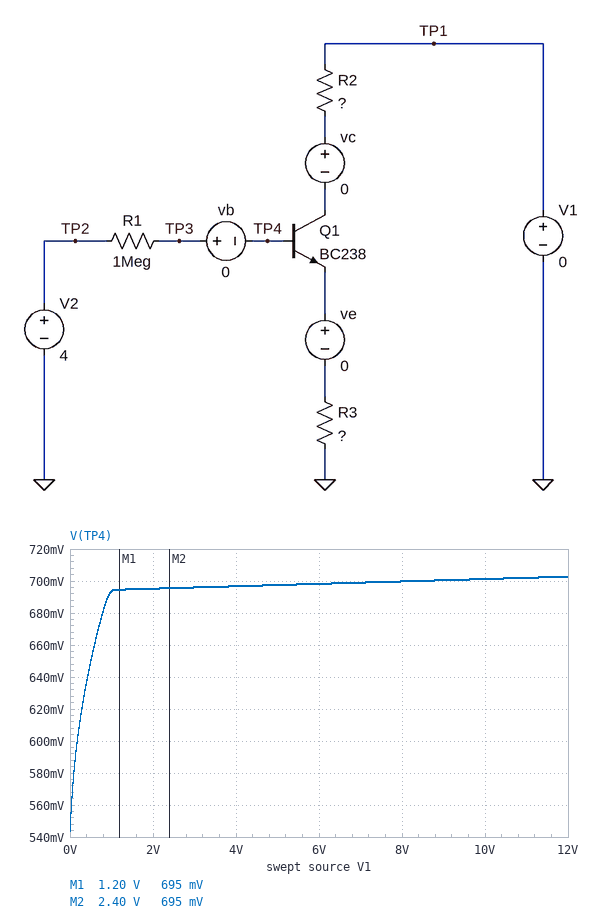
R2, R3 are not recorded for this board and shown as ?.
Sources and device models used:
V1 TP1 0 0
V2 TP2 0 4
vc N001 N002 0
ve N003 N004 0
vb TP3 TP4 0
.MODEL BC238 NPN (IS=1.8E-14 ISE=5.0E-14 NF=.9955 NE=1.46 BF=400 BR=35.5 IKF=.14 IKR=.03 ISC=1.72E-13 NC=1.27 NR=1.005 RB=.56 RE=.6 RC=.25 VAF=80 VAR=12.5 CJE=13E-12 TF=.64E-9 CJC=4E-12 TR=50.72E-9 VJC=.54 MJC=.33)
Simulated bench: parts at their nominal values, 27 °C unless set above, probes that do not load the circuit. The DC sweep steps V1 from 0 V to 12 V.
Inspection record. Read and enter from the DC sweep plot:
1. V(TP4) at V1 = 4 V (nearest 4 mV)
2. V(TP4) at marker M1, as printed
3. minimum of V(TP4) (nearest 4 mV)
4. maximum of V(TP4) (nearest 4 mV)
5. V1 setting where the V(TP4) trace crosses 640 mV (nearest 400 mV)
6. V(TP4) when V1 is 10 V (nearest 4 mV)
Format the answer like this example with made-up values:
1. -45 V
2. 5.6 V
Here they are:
1. 696 mV
2. 695 mV
3. 544 mV
4. 704 mV
5. 400 mV
6. 700 mV
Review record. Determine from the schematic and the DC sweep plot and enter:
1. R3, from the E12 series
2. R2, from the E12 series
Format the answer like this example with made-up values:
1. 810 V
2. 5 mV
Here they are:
1. 68 Ω
2. 820 Ω
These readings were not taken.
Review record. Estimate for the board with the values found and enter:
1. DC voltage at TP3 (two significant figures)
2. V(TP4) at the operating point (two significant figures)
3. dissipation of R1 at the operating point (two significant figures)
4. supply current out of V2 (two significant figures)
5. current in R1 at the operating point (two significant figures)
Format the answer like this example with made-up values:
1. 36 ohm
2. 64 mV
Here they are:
1. 540 mV
2. 540 mV
3. 12 µW
4. 3.5 µA
5. 3.5 µA
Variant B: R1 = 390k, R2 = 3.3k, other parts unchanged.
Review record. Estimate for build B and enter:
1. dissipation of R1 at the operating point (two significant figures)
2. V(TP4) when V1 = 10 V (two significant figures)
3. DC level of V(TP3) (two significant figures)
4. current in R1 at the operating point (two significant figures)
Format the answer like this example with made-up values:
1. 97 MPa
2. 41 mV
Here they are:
1. 30 µW
2. 820 mV
3. 570 mV
4. 8.8 µA
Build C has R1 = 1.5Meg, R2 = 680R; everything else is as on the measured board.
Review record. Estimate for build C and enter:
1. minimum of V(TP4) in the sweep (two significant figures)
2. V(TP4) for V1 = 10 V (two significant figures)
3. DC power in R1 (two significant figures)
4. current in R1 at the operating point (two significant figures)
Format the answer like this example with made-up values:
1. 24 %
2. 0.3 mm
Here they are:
1. 530 mV
2. 670 mV
3. 8.0 µW
4. 2.3 µA
